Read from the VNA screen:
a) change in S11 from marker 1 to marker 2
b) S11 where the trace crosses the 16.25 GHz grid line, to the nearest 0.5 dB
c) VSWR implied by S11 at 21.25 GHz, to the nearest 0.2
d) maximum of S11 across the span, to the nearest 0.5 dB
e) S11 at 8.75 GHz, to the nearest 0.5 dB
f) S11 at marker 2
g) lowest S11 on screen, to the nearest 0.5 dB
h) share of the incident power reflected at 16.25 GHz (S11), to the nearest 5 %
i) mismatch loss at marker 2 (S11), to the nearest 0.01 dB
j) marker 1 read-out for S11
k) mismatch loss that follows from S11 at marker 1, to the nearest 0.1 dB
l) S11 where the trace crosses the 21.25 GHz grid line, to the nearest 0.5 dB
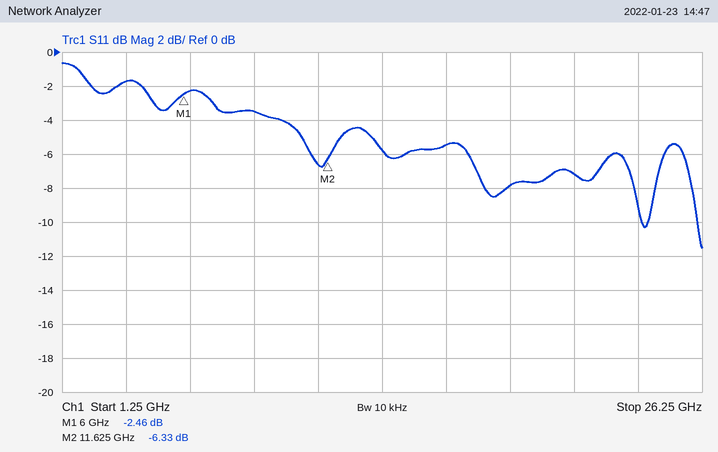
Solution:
-3.87 dB
-5.5 dB
2.6
-0.5 dB
-3.5 dB
-6.33 dB
-11.5 dB
30 %
1.15 dB
-2.46 dB
3.6 dB
-7.0 dB
